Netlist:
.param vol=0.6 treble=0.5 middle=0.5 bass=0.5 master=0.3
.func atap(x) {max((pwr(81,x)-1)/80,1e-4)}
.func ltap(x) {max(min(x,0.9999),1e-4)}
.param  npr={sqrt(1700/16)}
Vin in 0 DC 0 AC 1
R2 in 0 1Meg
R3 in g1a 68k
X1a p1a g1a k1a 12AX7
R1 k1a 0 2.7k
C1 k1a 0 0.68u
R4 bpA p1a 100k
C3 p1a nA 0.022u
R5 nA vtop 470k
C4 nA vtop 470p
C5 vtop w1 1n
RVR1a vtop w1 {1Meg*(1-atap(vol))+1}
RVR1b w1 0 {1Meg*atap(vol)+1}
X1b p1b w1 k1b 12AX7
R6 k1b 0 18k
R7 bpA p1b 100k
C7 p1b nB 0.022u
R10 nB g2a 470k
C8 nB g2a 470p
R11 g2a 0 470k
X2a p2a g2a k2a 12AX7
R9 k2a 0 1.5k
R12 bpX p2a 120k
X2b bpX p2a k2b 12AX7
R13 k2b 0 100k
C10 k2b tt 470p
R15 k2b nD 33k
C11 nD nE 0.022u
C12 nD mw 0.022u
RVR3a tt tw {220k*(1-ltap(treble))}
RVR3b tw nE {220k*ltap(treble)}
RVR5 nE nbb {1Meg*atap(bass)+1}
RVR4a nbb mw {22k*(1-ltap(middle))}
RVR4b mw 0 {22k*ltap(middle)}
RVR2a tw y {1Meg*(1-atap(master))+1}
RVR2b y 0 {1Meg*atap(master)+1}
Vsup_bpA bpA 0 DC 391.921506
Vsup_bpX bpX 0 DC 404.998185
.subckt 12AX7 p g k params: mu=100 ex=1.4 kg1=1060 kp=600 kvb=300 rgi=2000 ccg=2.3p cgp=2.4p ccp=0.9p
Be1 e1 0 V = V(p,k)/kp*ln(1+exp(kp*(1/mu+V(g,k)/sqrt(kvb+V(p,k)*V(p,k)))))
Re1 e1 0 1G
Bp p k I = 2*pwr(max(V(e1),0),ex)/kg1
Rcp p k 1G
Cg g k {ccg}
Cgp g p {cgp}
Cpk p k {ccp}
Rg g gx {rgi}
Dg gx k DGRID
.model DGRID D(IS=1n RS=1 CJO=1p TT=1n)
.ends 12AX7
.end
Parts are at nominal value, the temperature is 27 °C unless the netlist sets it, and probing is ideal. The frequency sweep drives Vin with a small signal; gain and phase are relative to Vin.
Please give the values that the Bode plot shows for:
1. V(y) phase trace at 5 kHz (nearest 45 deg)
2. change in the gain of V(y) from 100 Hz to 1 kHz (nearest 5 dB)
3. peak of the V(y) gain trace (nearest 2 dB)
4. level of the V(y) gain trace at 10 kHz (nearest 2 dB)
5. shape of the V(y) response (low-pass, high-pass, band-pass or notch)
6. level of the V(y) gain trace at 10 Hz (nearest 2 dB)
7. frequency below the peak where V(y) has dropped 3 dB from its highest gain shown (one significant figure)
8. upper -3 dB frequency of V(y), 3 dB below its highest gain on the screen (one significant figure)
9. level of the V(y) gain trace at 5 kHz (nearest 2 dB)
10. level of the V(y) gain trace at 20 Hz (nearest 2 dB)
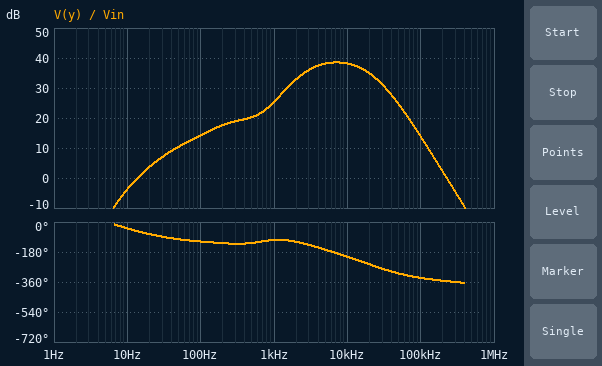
-180 deg
10 dB
38 dB
38 dB
band-pass
-4 dB
3 kHz
20 kHz
38 dB
4 dB
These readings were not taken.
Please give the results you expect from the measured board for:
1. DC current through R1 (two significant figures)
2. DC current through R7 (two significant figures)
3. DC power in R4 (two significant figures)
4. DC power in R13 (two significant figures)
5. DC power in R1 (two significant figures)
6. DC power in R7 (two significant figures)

940 µA
230 µA
88 mW
650 mW
2.4 mW
5.3 mW
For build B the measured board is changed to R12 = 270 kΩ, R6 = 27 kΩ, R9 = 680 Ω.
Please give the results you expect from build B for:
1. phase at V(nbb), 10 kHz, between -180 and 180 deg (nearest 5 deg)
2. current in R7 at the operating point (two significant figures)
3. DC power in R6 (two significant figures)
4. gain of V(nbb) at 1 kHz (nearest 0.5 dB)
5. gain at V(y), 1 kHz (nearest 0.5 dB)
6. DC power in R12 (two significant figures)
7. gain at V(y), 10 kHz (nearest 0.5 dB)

135 deg
160 µA
720 µW
53.5 dB
27.0 dB
280 mW
38.5 dB
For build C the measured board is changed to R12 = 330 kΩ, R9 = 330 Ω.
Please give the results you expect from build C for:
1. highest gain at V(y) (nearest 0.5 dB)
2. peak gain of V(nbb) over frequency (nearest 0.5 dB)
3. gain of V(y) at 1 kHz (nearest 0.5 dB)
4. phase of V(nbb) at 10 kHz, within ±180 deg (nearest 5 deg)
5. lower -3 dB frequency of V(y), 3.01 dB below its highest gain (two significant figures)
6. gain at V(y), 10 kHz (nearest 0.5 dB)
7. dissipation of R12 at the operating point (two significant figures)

43.5 dB
66.0 dB
31.5 dB
135 deg
2.5 kHz
42.5 dB
300 mW
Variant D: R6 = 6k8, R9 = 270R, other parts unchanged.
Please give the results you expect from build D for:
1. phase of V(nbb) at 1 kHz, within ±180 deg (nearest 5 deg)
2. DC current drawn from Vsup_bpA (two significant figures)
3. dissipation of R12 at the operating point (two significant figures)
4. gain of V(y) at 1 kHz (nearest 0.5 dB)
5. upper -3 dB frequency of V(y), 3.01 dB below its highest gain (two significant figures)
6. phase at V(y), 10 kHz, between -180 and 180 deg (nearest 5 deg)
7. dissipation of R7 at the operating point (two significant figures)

-115 deg
1.4 mA
500 mW
37.5 dB
16 kHz
145 deg
25 mW
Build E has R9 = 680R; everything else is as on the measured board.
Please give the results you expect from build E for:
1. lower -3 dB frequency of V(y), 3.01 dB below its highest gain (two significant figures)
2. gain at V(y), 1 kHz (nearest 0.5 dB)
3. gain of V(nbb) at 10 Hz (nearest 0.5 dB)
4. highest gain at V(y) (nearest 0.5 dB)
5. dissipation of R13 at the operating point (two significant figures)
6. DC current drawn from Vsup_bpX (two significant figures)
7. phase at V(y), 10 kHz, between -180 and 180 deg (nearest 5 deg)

2.7 kHz
28.0 dB
17.5 dB
41.0 dB
420 mW
3.7 mA
145 deg
